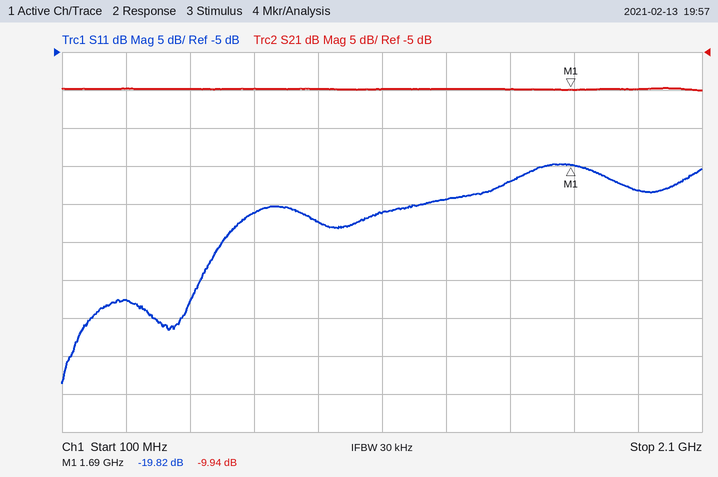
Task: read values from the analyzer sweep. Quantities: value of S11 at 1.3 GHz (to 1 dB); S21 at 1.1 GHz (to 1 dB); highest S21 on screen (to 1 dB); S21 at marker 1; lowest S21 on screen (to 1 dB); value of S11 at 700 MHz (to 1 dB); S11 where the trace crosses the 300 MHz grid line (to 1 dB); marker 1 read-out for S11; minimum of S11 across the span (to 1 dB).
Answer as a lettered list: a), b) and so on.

a) -24 dB
b) -10 dB
c) -10 dB
d) -9.94 dB
e) -10 dB
f) -26 dB
g) -38 dB
h) -19.82 dB
i) -49 dB
